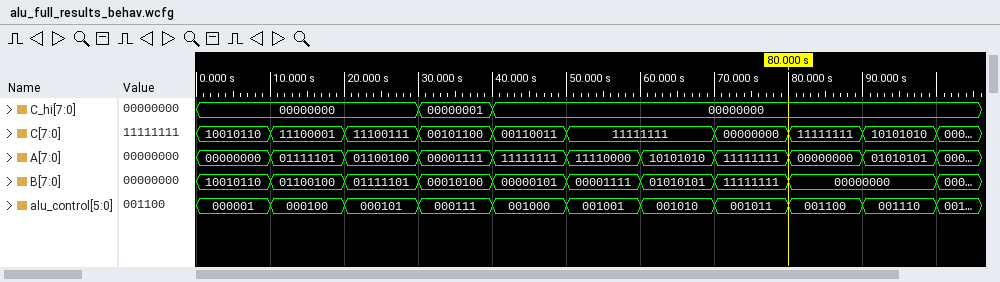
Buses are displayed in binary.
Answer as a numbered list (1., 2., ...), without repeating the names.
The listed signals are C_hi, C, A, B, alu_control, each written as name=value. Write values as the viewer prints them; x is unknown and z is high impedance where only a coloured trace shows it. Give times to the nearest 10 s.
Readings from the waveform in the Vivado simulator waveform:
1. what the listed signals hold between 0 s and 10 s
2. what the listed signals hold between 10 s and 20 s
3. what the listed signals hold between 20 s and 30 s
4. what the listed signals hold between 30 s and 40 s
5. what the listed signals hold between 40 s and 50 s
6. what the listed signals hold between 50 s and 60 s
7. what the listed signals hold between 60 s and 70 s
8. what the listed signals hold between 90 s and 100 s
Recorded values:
1. C_hi=00000000, C=10010110, A=00000000, B=10010110, alu_control=000001
2. C_hi=00000000, C=11100001, A=01111101, B=01100100, alu_control=000100
3. C_hi=00000000, C=11100111, A=01100100, B=01111101, alu_control=000101
4. C_hi=00000001, C=00101100, A=00001111, B=00010100, alu_control=000111
5. C_hi=00000000, C=00110011, A=11111111, B=00000101, alu_control=001000
6. C_hi=00000000, C=11111111, A=11110000, B=00001111, alu_control=001001
7. C_hi=00000000, C=11111111, A=10101010, B=01010101, alu_control=001010
8. C_hi=00000000, C=10101010, A=01010101, B=00000000, alu_control=001110
